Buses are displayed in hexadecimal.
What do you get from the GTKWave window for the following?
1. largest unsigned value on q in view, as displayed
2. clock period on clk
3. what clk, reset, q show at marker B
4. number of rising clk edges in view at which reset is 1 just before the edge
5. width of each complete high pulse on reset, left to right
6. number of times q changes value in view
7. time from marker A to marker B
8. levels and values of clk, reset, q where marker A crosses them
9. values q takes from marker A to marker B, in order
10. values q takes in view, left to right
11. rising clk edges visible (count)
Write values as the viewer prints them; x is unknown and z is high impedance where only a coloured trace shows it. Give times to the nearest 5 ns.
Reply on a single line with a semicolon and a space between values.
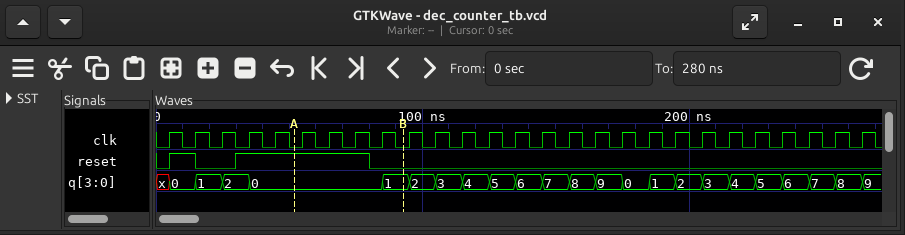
9; 10 ns; clk=0, reset=0, q=1; 6; 10 ns, 50 ns; 23; 40 ns; clk=0, reset=1, q=0; 0, 1; x, 0, 1, 2, 0, 1, 2, 3, 4, 5, 6, 7, 8, 9, 0, 1, 2, 3, 4, 5, 6, 7, 8, 9; 27
